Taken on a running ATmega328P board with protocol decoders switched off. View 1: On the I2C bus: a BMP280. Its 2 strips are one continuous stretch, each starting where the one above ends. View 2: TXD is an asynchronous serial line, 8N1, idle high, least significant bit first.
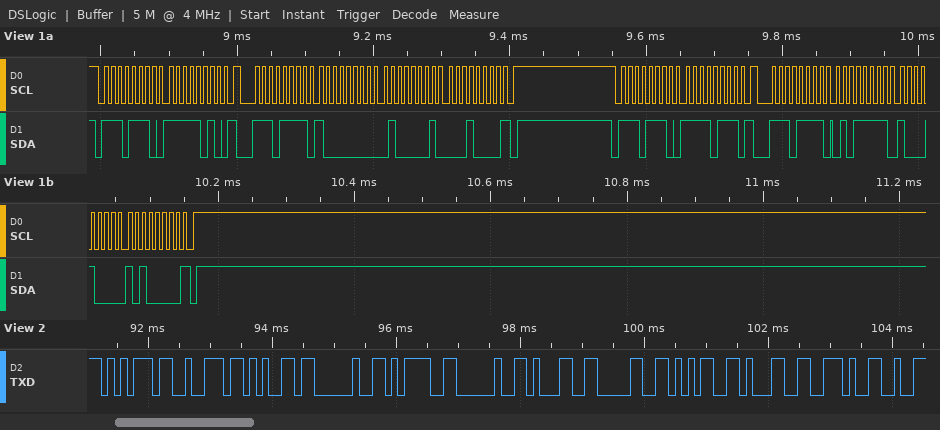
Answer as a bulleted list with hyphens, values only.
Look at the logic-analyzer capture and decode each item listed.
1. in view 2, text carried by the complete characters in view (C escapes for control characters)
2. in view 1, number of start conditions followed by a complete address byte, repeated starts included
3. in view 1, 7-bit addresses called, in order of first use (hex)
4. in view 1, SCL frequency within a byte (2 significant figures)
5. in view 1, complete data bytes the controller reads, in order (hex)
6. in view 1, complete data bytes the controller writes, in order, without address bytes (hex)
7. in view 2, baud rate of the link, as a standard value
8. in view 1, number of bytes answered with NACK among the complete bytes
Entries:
- "ure = 1051."
- 4
- 0x77
- 100 kHz
- 80 41 10 5F 88 A0
- FA F7
- 9600 baud
- 2
